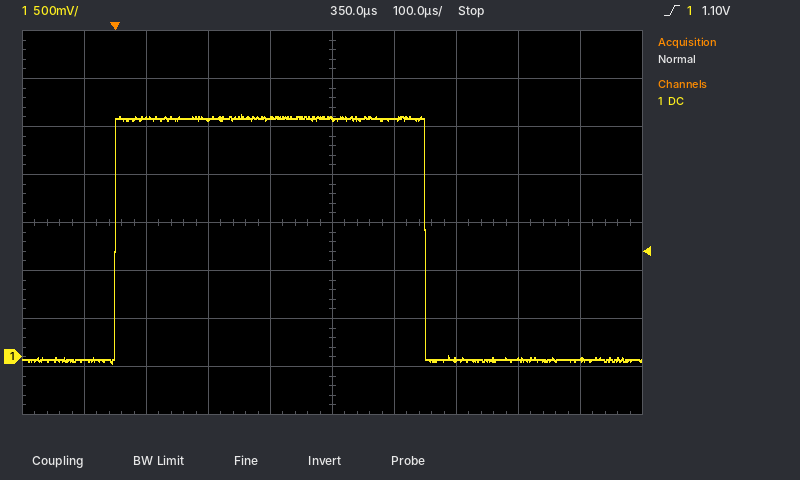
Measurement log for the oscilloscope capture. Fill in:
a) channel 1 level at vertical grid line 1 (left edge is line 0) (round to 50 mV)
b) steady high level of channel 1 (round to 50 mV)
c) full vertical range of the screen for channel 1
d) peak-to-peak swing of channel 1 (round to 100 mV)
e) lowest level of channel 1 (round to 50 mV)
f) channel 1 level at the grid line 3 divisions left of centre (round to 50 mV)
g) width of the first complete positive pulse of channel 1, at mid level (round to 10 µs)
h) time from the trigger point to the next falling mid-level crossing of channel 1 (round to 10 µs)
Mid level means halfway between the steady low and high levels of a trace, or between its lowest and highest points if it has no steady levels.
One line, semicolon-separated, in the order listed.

-50 mV; 2.50 V; 4 V; 2.60 V; -50 mV; 2.50 V; 500 µs; 500 µs
